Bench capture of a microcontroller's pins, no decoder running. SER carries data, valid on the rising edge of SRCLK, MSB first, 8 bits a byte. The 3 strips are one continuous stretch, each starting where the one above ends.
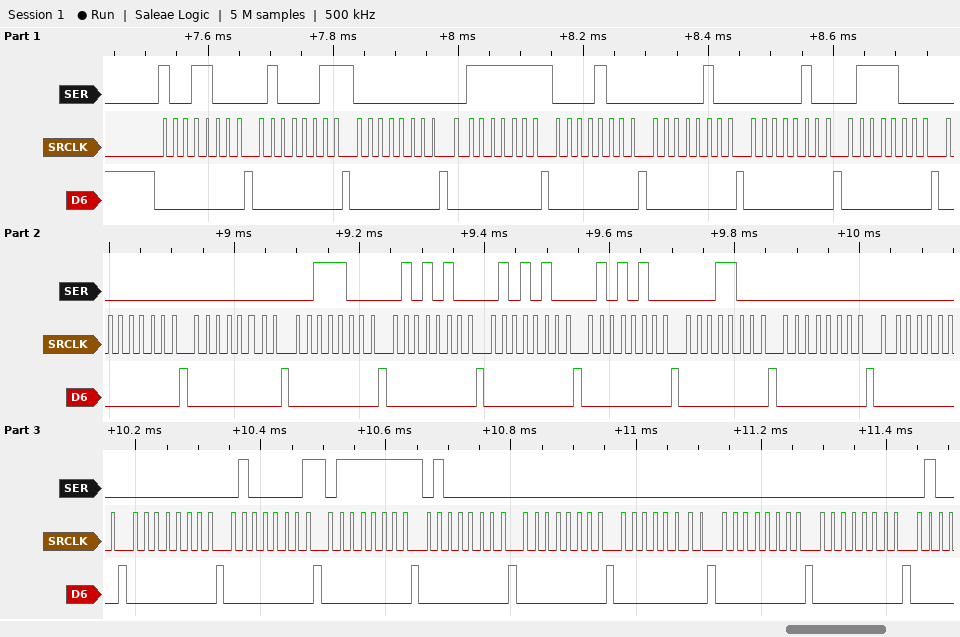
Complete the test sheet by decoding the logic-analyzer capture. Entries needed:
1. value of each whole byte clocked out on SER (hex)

0x98 0x43 0x00 0x7F 0x08 0x04 0x04 0x78 0x00 0x00 0x38 0x54 0x54 0x54 0x18 0x00 0x00 0x00 0x41 0x7F 0x40 0x00 0x00 0x00 0x00
